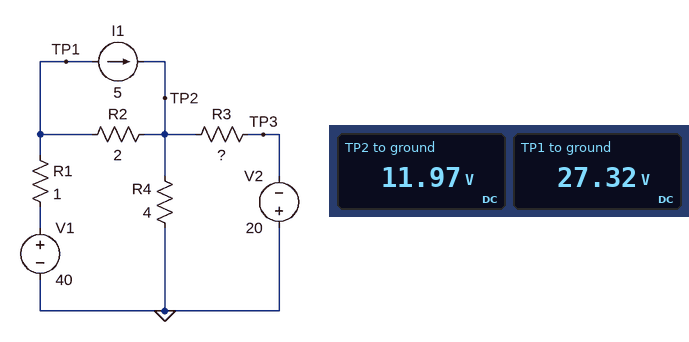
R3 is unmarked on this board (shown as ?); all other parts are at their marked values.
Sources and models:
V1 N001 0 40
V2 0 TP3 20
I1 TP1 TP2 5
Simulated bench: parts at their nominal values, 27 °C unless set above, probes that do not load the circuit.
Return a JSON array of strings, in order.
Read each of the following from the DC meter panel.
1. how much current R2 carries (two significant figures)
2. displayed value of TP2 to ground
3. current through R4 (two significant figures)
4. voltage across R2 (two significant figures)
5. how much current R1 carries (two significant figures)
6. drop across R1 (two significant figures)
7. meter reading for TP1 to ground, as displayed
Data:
["7.7 A", "11.97 V", "3.0 A", "15 V", "13 A", "13 V", "27.32 V"]
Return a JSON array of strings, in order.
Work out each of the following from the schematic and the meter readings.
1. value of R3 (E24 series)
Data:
["3.3 Ω"]
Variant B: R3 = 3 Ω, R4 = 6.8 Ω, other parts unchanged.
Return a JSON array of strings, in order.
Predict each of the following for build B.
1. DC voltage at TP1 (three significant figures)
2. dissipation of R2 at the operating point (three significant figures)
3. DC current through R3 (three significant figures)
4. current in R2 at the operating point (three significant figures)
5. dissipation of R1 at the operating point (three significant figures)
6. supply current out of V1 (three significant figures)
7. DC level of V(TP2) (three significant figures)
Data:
["27.4 V", "115 W", "10.8 A", "7.57 A", "158 W", "12.6 A", "12.3 V"]
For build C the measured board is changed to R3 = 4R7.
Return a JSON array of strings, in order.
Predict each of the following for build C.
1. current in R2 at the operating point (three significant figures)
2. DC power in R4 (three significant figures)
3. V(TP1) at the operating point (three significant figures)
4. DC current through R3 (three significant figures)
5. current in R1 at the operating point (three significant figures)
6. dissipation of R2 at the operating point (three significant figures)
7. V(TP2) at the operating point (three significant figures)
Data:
["6.47 A", "60.8 W", "28.5 V", "7.57 A", "11.5 A", "83.7 W", "15.6 V"]
